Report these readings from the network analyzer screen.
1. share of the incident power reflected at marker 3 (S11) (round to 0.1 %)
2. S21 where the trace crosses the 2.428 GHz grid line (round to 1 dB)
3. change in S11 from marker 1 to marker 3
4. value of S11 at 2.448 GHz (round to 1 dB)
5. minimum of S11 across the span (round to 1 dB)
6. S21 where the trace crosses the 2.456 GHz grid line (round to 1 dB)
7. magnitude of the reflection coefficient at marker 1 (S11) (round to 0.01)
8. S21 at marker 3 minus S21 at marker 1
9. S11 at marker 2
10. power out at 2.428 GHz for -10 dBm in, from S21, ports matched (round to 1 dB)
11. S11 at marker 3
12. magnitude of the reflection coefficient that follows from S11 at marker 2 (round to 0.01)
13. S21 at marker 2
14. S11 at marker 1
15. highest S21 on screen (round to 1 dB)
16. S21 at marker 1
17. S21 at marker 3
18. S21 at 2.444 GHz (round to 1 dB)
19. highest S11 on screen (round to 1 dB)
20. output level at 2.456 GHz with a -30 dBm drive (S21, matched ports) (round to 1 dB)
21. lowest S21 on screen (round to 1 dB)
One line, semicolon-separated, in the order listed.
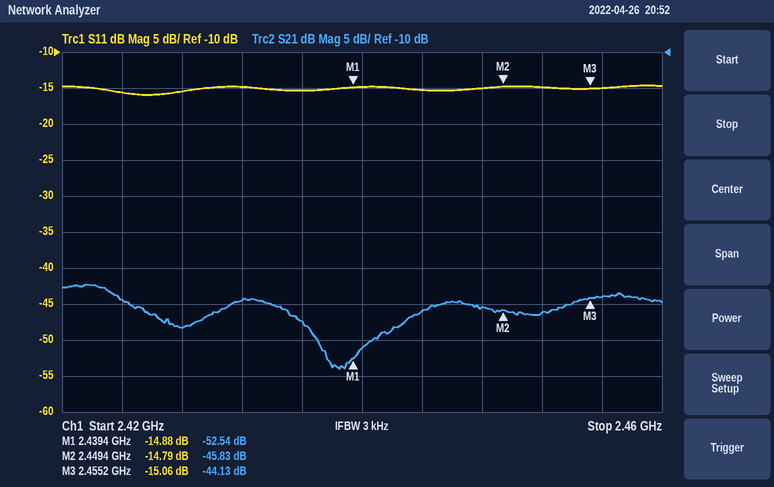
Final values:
3.1 %; -48 dB; -0.18 dB; -15 dB; -16 dB; -44 dB; 0.18; 8.41 dB; -14.79 dB; -58 dBm; -15.06 dB; 0.18; -45.83 dB; -14.88 dB; -42 dB; -52.54 dB; -44.13 dB; -46 dB; -15 dB; -74 dBm; -54 dB
